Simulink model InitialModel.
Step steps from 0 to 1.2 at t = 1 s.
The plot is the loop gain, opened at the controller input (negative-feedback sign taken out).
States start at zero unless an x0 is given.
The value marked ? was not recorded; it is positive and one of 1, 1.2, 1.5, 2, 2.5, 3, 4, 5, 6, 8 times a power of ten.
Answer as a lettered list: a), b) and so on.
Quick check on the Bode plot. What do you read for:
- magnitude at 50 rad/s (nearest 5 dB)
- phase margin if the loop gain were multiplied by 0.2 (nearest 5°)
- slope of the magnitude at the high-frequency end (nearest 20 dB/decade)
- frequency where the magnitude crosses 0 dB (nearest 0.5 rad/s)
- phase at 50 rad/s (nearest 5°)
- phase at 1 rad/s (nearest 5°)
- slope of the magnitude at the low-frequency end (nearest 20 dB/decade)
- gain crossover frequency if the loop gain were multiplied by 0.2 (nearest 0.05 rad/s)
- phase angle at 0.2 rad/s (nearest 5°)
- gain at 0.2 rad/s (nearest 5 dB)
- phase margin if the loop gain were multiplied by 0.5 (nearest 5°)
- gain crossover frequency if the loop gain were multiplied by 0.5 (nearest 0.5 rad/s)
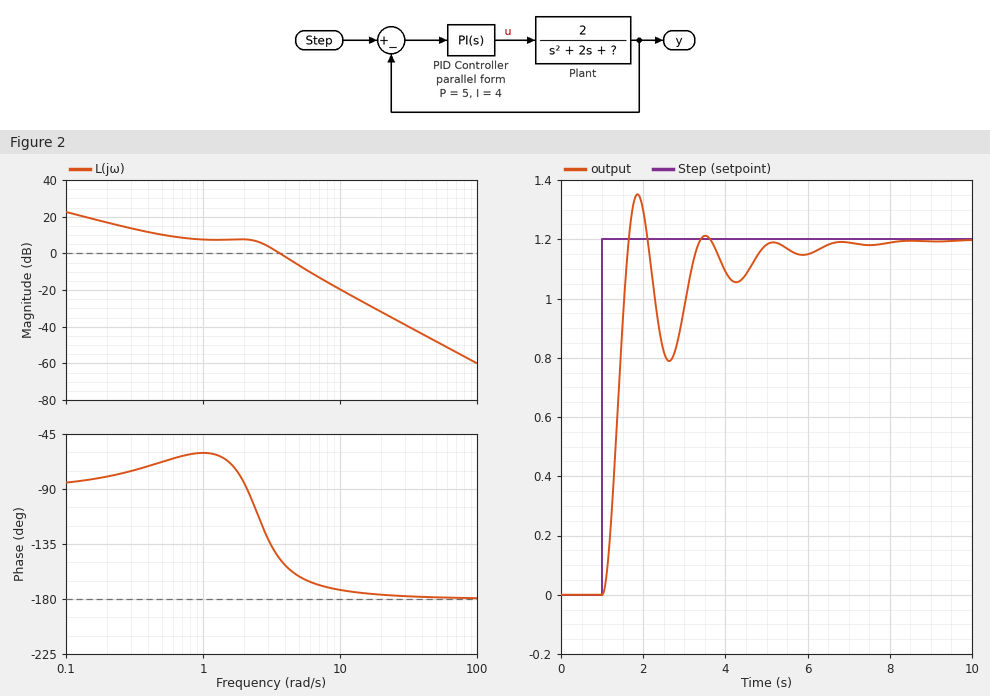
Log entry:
a) -50 dB
b) 105°
c) -40 dB/decade
d) 3.5 rad/s
e) -180°
f) -60°
g) -20 dB/decade
h) 0.30 rad/s
i) -80°
j) 15 dB
k) 65°
l) 2.5 rad/s
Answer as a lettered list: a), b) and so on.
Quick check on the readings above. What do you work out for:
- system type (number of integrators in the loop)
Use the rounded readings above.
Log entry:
a) 1
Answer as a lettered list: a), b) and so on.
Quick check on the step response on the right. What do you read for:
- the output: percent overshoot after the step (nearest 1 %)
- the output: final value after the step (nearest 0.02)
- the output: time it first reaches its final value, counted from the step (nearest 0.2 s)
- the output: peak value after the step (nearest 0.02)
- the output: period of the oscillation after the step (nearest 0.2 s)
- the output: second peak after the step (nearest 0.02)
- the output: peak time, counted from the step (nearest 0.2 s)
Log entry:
a) 13 %
b) 1.20
c) 0.6 s
d) 1.36
e) 1.6 s
f) 1.22
g) 0.8 s
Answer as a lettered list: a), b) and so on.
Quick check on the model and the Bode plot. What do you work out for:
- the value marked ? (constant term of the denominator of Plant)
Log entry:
a) 6
